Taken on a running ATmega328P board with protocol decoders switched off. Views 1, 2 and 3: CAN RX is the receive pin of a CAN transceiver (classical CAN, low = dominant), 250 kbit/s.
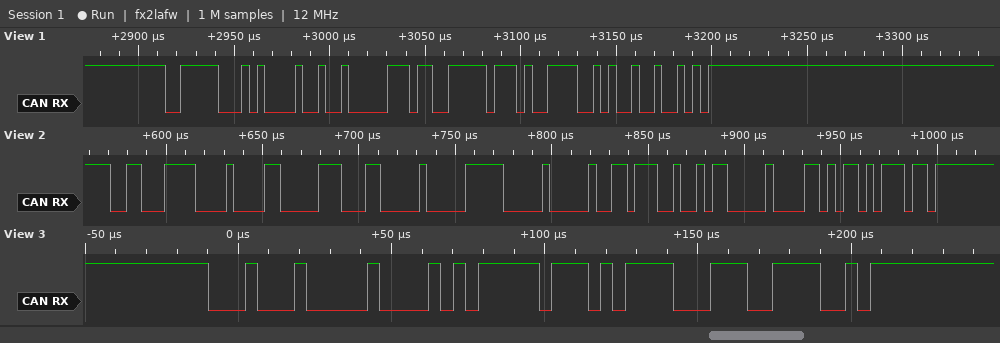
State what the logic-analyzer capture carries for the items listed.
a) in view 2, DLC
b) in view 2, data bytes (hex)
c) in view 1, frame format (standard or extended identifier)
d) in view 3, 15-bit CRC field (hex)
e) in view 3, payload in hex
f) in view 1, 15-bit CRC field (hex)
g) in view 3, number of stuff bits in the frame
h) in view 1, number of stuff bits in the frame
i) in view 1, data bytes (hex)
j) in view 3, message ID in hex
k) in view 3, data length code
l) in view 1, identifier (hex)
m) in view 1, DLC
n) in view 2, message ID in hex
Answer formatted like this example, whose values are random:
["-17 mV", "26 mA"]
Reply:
["8", "60 C6 00 78 00 DC 96 00", "standard", "0x473C", "BF D7", "0x1492", "2", "3", "90 6C FF 4F", "0x110", "2", "0x3E5", "4", "0x31E"]
